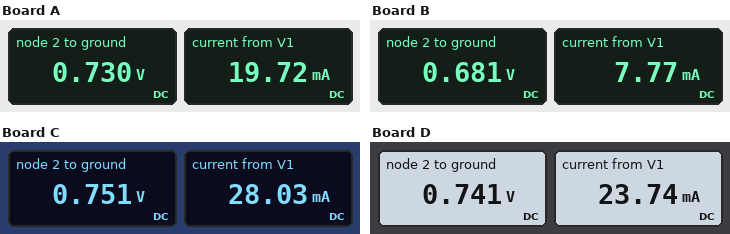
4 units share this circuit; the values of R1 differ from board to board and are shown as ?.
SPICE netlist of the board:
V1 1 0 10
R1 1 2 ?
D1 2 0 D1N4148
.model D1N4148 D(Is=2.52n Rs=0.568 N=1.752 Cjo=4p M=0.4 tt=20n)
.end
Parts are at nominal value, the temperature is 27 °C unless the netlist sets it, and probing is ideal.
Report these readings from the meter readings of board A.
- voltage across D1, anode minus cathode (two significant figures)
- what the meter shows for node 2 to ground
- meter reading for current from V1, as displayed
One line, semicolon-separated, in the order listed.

730 mV; 0.730 V; 19.72 mA
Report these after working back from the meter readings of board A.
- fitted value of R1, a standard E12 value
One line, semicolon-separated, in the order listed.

470 Ω
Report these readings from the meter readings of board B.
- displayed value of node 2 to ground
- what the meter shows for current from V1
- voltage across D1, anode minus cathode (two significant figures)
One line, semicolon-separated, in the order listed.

0.681 V; 7.77 mA; 680 mV
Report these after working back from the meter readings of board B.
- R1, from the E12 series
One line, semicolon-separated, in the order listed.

1.2 kΩ
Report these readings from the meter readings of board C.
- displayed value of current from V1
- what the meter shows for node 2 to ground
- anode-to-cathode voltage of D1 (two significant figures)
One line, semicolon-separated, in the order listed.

28.03 mA; 0.751 V; 750 mV
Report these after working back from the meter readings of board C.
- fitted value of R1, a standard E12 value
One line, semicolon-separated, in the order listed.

330 Ω
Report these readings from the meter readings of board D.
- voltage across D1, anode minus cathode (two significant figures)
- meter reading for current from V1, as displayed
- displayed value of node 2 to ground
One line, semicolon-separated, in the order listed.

740 mV; 23.74 mA; 0.741 V
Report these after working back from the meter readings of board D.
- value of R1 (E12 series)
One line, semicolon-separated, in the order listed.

390 Ω
